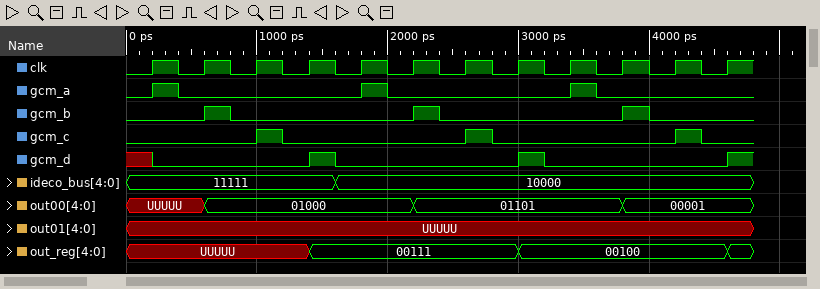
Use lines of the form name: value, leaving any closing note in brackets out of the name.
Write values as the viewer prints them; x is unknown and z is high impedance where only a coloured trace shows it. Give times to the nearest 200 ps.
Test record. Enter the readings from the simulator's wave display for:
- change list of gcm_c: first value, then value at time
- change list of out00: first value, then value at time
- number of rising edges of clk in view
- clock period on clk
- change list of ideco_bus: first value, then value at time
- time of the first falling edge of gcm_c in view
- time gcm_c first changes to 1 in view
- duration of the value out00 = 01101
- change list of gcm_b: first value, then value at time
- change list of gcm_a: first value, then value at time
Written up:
change list of gcm_c: first value, then value at time: 0, 1 at 1000 ps, 0 at 1200 ps, 1 at 2600 ps, 0 at 2800 ps, 1 at 4200 ps, 0 at 4400 ps
change list of out00: first value, then value at time: UUUUU, 01000 at 600 ps, 01101 at 2200 ps, 00001 at 3800 ps
number of rising edges of clk in view: 12
clock period on clk: 400 ps
change list of ideco_bus: first value, then value at time: 11111, 10000 at 1600 ps
time of the first falling edge of gcm_c in view: 1200 ps
time gcm_c first changes to 1 in view: 1000 ps
duration of the value out00 = 01101: 1600 ps
change list of gcm_b: first value, then value at time: 0, 1 at 600 ps, 0 at 800 ps, 1 at 2200 ps, 0 at 2400 ps, 1 at 3800 ps, 0 at 4000 ps
change list of gcm_a: first value, then value at time: 0, 1 at 200 ps, 0 at 400 ps, 1 at 1800 ps, 0 at 2000 ps, 1 at 3400 ps, 0 at 3600 ps
